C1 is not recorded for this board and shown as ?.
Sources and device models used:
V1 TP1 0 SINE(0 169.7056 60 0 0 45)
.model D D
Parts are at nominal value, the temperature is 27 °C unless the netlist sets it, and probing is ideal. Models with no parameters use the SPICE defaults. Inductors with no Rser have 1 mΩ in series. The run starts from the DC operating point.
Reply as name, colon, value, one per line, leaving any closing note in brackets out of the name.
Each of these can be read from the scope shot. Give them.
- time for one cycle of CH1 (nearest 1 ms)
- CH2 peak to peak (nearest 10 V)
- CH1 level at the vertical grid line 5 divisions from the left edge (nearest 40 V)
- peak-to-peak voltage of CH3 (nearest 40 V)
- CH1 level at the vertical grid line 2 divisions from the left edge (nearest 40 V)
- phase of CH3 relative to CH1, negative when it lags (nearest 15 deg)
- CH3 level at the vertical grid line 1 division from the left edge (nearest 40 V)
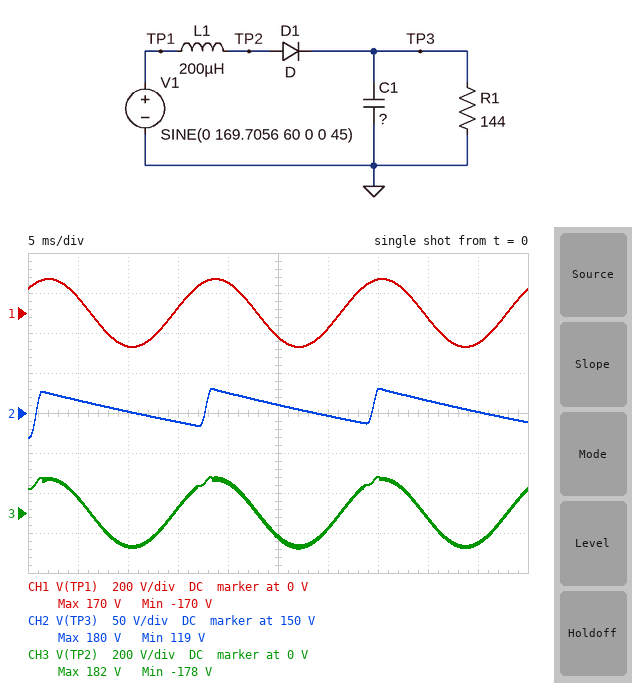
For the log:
time for one cycle of CH1: 17 ms
CH2 peak to peak: 60 V
CH1 level at the vertical grid line 5 divisions from the left edge: -120 V
peak-to-peak voltage of CH3: 360 V
CH1 level at the vertical grid line 2 divisions from the left edge: -160 V
phase of CH3 relative to CH1, negative when it lags: 0 deg
CH3 level at the vertical grid line 1 division from the left edge: 80 V
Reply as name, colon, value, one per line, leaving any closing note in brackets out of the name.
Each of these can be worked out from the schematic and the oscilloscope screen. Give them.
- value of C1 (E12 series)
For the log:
value of C1: 390 µF
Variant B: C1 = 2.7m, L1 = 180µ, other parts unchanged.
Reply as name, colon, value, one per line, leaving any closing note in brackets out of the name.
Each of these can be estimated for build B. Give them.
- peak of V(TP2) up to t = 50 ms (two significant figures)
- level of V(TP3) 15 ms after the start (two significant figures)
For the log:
peak of V(TP2) up to t = 50 ms: 210 V
level of V(TP3) 15 ms after the start: 200 V
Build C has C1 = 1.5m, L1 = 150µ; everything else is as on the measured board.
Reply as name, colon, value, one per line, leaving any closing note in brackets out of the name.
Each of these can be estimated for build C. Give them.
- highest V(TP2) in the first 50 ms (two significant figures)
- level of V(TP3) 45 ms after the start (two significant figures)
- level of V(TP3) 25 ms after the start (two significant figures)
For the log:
highest V(TP2) in the first 50 ms: 200 V
level of V(TP3) 45 ms after the start: 160 V
level of V(TP3) 25 ms after the start: 180 V
